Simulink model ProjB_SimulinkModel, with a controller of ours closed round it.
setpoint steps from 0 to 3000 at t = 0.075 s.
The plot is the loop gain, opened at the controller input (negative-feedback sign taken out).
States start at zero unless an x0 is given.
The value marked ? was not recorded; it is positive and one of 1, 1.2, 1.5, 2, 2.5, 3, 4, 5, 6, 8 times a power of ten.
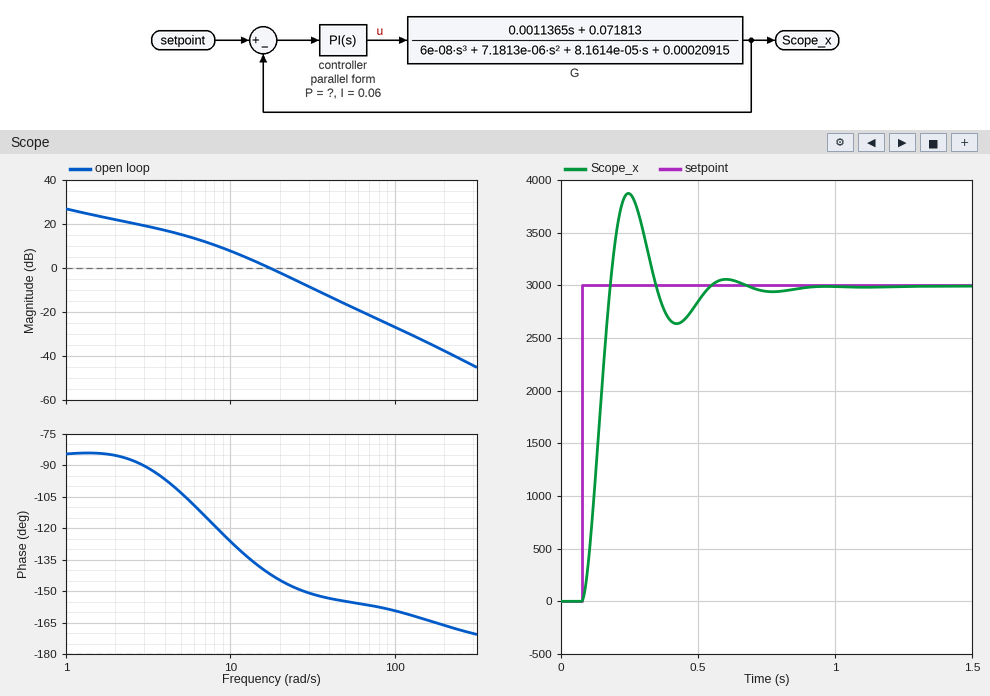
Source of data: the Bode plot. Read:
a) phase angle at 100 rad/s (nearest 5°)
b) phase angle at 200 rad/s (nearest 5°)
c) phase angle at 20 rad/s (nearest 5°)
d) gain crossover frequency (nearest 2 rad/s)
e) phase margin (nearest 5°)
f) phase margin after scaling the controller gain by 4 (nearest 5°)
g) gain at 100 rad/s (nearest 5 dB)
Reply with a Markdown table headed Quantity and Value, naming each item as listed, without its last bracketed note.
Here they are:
| Quantity | Value |
|---|---|
| phase angle at 100 rad/s | -160° |
| phase angle at 200 rad/s | -165° |
| phase angle at 20 rad/s | -145° |
| gain crossover frequency | 18 rad/s |
| phase margin | 40° |
| phase margin after scaling the controller gain by 4 | 25° |
| gain at 100 rad/s | -25 dB |
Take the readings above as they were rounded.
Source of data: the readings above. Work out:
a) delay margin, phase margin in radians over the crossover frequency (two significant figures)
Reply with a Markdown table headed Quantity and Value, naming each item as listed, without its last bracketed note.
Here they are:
| Quantity | Value |
|---|---|
| delay margin, phase margin in radians over the crossover frequency | 0.039 s |
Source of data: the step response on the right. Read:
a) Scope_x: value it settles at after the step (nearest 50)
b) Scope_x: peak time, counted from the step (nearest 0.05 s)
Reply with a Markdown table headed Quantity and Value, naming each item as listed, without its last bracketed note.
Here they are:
| Quantity | Value |
|---|---|
| Scope_x: value it settles at after the step | 3000 |
| Scope_x: peak time, counted from the step | 0.15 s |
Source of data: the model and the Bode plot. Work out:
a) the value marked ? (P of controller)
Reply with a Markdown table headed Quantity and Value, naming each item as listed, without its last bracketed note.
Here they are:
| Quantity | Value |
|---|---|
| the value marked ? | 0.03 |
